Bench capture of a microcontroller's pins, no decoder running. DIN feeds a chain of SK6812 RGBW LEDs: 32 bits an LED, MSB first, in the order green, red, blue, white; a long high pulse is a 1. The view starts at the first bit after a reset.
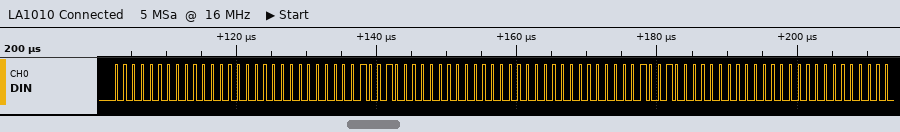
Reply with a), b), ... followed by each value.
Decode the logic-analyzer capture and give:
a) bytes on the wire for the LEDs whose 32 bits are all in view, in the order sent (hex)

a) 00 00 00 09 00 00 00 09
